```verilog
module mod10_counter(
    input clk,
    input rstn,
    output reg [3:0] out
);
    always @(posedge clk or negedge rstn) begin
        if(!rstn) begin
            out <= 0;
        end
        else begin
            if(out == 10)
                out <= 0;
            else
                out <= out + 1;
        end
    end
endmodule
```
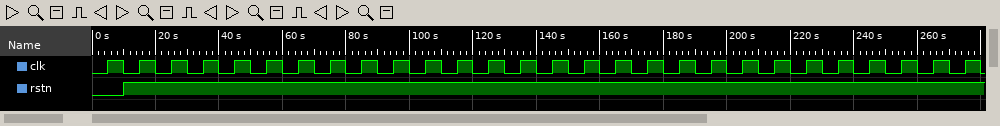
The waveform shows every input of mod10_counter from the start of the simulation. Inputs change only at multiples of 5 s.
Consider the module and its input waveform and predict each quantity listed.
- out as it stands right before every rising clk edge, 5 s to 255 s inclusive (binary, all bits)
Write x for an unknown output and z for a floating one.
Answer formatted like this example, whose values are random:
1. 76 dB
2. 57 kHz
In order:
1. 0000, 0000, 0001, 0010, 0011, 0100, 0101, 0110, 0111, 1000, 1001, 1010, 0000, 0001, 0010, 0011, 0100, 0101, 0110, 0111, 1000, 1001, 1010, 0000, 0001, 0010
